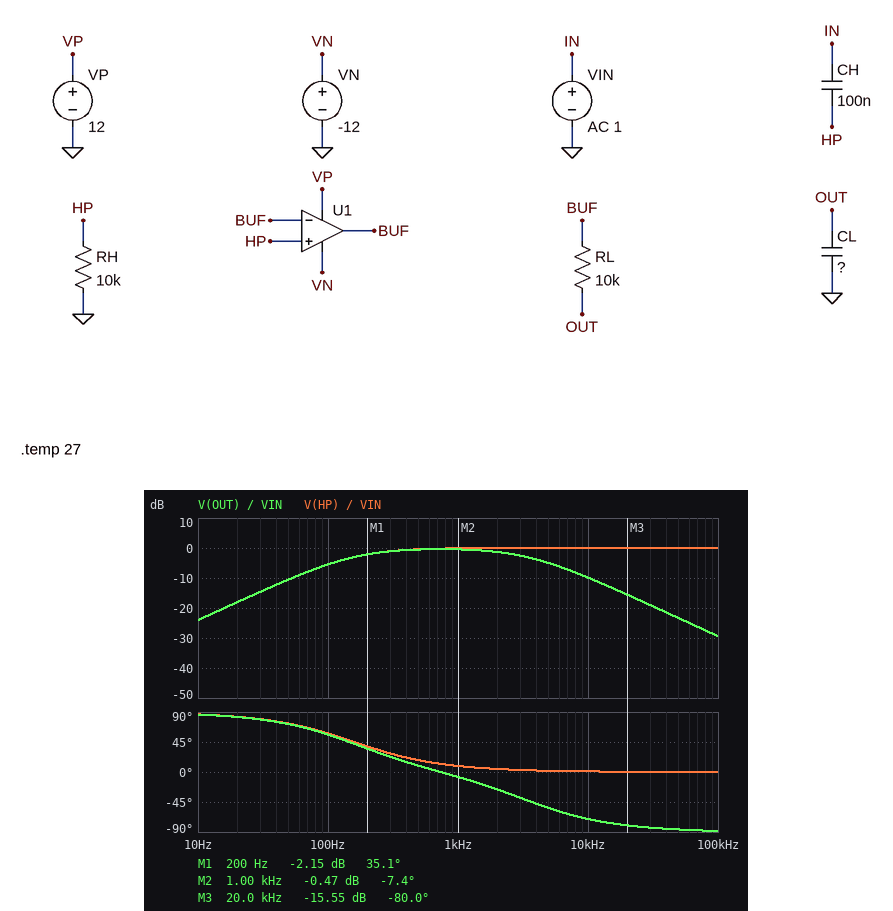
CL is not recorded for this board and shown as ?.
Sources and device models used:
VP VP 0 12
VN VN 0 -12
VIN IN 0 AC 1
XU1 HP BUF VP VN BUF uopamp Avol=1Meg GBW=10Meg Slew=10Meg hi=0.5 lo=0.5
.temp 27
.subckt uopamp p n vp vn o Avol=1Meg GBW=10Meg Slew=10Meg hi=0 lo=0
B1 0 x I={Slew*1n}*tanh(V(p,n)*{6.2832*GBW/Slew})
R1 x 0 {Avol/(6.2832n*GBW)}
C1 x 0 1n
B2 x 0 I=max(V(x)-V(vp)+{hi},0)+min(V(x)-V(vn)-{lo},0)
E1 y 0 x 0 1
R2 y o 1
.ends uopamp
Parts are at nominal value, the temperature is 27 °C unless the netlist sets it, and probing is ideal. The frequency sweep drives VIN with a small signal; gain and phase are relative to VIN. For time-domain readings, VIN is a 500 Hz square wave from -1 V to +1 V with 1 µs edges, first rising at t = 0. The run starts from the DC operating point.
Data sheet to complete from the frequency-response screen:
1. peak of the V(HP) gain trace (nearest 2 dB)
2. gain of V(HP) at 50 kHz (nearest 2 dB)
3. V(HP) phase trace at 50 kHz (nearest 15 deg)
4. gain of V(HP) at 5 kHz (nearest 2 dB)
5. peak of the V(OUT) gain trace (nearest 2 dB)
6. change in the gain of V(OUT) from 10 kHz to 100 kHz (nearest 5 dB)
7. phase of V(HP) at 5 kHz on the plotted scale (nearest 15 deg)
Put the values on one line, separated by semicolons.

0 dB; 0 dB; 0 deg; 0 dB; 0 dB; -20 dB; 0 deg
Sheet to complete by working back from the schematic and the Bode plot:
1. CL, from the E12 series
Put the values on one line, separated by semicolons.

4.7 nF
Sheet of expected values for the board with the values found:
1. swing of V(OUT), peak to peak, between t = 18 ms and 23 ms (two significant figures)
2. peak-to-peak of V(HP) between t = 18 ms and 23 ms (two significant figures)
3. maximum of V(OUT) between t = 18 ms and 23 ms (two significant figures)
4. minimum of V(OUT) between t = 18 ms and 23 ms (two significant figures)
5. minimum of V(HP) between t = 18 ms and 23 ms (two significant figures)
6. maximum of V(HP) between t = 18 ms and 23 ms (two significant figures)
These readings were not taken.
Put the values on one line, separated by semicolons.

2.5 V; 2.9 V; 1.2 V; -1.2 V; -1.5 V; 1.5 V
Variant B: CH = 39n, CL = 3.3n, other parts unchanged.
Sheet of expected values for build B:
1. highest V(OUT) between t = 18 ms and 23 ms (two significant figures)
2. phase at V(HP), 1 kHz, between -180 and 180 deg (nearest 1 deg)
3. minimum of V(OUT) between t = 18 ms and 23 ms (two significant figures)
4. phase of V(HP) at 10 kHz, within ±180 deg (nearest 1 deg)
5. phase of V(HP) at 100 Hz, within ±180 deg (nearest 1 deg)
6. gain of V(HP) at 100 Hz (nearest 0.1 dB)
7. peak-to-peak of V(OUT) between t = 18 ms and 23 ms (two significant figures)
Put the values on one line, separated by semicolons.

1.5 V; 22 deg; -1.5 V; 2 deg; 76 deg; -12.5 dB; 2.9 V
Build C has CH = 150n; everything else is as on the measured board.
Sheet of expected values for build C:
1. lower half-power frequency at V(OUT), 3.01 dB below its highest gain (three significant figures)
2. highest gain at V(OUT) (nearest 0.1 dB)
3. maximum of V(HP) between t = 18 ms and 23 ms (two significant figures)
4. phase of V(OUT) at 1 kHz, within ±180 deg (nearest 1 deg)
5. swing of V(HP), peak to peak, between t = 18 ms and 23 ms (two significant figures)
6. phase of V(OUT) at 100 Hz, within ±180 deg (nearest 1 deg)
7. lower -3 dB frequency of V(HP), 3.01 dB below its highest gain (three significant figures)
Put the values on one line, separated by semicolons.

100 Hz; -0.3 dB; 1.3 V; -10 deg; 2.6 V; 45 deg; 106 Hz
